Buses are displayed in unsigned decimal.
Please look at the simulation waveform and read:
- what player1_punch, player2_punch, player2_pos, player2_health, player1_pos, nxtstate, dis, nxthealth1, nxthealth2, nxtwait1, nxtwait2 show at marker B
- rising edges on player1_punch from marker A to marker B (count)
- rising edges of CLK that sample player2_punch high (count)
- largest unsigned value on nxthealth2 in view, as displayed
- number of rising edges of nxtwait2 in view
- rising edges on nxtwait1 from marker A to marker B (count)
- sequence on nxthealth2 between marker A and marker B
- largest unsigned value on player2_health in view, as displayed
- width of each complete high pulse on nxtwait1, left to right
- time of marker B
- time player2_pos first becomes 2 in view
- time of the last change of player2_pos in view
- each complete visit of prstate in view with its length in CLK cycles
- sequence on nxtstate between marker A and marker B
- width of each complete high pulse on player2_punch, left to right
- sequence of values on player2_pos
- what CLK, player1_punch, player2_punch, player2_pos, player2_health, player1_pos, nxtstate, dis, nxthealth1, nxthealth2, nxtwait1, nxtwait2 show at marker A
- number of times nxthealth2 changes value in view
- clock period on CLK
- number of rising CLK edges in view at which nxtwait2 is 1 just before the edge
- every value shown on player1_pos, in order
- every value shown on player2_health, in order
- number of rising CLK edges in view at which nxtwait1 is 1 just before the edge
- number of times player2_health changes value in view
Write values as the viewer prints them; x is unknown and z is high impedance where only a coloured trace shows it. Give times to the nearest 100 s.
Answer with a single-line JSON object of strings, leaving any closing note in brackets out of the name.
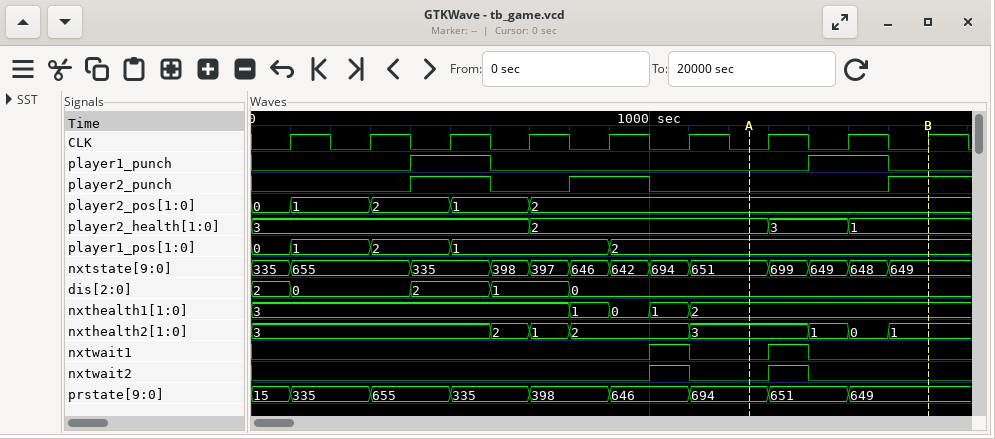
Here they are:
{"what player1_punch, player2_punch, player2_pos, player2_health, player1_pos, nxtstate, dis, nxthealth1, nxthealth2, nxtwait1, nxtwait2 show at marker B": "player1_punch=0, player2_punch=1, player2_pos=2, player2_health=1, player1_pos=2, nxtstate=649, dis=0, nxthealth1=2, nxthealth2=1, nxtwait1=0, nxtwait2=0", "rising edges on player1_punch from marker A to marker B": "1", "rising edges of CLK that sample player2_punch high": "3", "largest unsigned value on nxthealth2 in view, as displayed": "3", "number of rising edges of nxtwait2 in view": "2", "rising edges on nxtwait1 from marker A to marker B": "1", "sequence on nxthealth2 between marker A and marker B": "3, 1, 0, 1", "largest unsigned value on player2_health in view, as displayed": "3", "width of each complete high pulse on nxtwait1, left to right": "100 s, 100 s", "time of marker B": "1700 s", "time player2_pos first becomes 2 in view": "300 s", "time of the last change of player2_pos in view": "700 s", "each complete visit of prstate in view with its length in CLK cycles": "335: 1, 655: 1, 335: 1, 398: 1, 646: 1, 694: 1, 651: 1", "sequence on nxtstate between marker A and marker B": "651, 699, 649, 648, 649", "width of each complete high pulse on player2_punch, left to right": "200 s, 200 s", "sequence of values on player2_pos": "0, 1, 2, 1, 2", "what CLK, player1_punch, player2_punch, player2_pos, player2_health, player1_pos, nxtstate, dis, nxthealth1, nxthealth2, nxtwait1, nxtwait2 show at marker A": "CLK=0, player1_punch=0, player2_punch=0, player2_pos=2, player2_health=2, player1_pos=2, nxtstate=651, dis=0, nxthealth1=2, nxthealth2=3, nxtwait1=0, nxtwait2=0", "number of times nxthealth2 changes value in view": "7", "clock period on CLK": "200 s", "number of rising CLK edges in view at which nxtwait2 is 1 just before the edge": "1", "every value shown on player1_pos, in order": "0, 1, 2, 1, 2", "every value shown on player2_health, in order": "3, 2, 3, 1", "number of rising CLK edges in view at which nxtwait1 is 1 just before the edge": "1", "number of times player2_health changes value in view": "3"}
